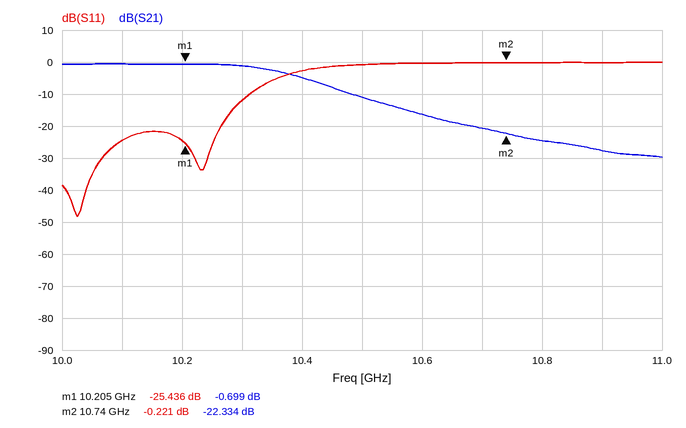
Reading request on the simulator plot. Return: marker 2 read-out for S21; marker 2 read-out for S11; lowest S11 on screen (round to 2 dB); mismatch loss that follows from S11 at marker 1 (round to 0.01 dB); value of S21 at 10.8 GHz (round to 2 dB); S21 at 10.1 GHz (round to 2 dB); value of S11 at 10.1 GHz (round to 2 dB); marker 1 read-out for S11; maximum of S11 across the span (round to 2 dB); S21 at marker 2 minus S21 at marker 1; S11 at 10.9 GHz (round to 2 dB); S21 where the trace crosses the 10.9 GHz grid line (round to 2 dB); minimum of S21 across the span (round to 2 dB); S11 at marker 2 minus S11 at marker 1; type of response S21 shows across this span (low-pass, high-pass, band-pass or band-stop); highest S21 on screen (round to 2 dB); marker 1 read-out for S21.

-22.334 dB
-0.221 dB
-48 dB
0.01 dB
-24 dB
0 dB
-24 dB
-25.436 dB
0 dB
-21.635 dB
0 dB
-28 dB
-30 dB
25.215 dB
low-pass
0 dB
-0.699 dB
